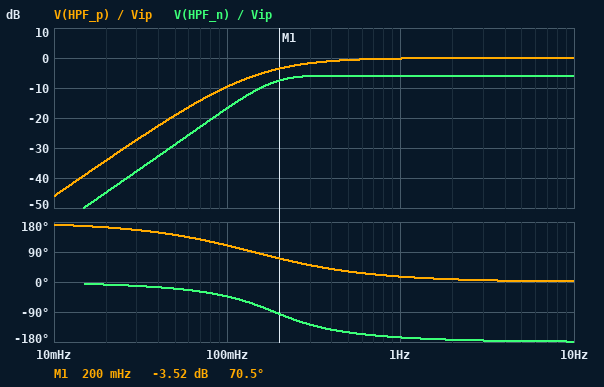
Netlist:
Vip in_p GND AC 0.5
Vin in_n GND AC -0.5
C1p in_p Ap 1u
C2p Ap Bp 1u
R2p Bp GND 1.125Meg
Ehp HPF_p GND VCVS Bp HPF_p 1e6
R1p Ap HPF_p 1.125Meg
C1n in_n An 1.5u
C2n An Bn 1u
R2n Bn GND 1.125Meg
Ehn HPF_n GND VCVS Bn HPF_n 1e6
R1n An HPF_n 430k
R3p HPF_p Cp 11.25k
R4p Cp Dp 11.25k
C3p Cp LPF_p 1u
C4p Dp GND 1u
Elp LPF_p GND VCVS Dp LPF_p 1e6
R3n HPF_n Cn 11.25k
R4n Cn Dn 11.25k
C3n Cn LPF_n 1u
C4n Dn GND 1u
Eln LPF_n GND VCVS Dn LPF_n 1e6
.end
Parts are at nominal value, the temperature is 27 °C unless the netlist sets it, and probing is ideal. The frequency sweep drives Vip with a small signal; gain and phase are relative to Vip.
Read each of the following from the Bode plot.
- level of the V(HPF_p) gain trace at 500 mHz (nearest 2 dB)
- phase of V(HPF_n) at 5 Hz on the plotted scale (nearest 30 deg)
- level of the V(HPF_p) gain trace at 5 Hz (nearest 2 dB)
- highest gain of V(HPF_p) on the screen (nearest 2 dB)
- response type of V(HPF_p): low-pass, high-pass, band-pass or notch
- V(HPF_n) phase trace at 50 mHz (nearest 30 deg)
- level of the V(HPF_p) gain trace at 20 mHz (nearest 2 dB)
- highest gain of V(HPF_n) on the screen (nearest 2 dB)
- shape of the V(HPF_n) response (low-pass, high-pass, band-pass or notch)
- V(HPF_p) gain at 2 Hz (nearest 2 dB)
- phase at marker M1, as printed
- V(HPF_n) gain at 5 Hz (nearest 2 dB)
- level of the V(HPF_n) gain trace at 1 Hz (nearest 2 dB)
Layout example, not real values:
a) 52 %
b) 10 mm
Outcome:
a) 0 dB
b) -180 deg
c) 0 dB
d) 0 dB
e) high-pass
f) -30 deg
g) -34 dB
h) -6 dB
i) high-pass
j) 0 dB
k) 70.5 deg
l) -6 dB
m) -6 dB
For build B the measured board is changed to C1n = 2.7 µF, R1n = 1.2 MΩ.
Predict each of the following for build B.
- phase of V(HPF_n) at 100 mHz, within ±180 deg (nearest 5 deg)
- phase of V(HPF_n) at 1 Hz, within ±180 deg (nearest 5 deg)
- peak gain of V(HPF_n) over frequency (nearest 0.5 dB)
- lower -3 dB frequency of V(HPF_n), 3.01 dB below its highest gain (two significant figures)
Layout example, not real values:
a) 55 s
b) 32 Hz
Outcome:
a) -100 deg
b) -170 deg
c) -6.0 dB
d) 160 mHz
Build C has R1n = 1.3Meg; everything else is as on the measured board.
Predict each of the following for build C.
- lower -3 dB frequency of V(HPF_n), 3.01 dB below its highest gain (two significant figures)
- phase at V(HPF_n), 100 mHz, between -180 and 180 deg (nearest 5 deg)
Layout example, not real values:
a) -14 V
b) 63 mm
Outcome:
a) 190 mHz
b) -85 deg
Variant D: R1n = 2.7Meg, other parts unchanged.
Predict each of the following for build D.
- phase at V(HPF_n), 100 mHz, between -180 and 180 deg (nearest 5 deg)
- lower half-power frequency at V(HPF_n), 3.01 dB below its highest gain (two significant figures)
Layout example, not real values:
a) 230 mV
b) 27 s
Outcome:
a) -100 deg
b) 210 mHz
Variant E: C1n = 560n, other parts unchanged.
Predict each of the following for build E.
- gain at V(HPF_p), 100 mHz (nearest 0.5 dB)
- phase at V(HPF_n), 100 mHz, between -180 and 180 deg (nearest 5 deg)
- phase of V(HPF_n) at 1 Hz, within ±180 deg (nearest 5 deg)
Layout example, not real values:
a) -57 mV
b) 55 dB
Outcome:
a) -9.5 dB
b) -25 deg
c) -155 deg
